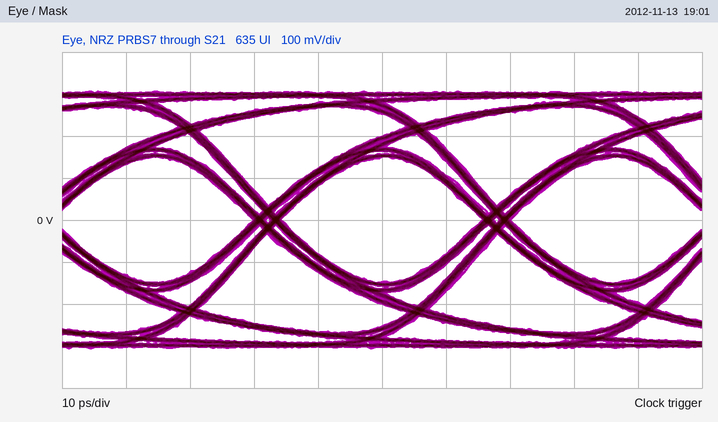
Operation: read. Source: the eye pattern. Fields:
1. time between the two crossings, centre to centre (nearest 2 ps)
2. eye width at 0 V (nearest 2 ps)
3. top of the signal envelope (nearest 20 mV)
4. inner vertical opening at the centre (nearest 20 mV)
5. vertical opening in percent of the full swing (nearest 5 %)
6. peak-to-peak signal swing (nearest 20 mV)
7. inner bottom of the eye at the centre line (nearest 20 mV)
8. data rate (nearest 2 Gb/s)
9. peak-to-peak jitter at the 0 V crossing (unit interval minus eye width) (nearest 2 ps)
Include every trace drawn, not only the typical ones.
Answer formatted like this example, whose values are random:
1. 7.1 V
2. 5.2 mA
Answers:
1. 36 ps
2. 32 ps
3. 300 mV
4. 300 mV
5. 50 %
6. 620 mV
7. -140 mV
8. 28 Gb/s
9. 4 ps
